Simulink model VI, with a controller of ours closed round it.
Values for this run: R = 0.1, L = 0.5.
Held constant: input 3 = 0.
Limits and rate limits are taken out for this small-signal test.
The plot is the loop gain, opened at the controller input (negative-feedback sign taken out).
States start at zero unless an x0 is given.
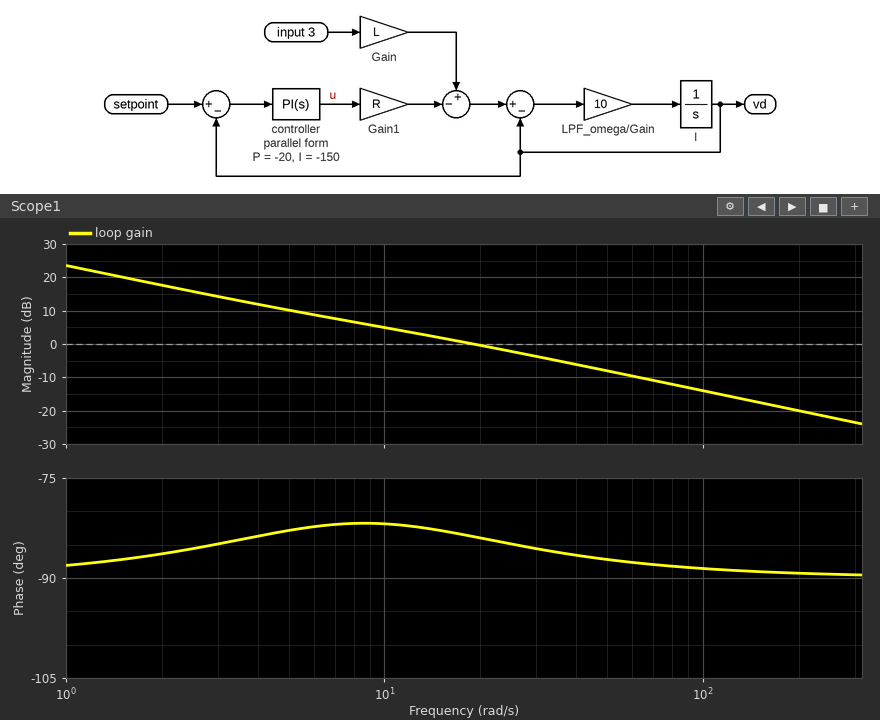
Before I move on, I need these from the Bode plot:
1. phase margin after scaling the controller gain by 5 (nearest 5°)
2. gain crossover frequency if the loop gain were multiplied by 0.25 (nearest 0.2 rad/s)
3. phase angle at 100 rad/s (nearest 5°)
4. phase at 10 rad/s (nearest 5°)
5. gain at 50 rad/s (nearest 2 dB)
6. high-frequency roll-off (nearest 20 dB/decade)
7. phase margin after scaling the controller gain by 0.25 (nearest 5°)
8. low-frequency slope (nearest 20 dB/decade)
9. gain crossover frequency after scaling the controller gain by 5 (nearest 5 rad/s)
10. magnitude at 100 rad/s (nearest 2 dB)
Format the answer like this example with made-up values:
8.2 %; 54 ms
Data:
90°; 4.0 rad/s; -90°; -80°; -8 dB; -20 dB/decade; 95°; -20 dB/decade; 100 rad/s; -14 dB
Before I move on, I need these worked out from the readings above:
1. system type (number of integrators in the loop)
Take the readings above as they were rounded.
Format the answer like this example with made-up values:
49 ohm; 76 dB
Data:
1
